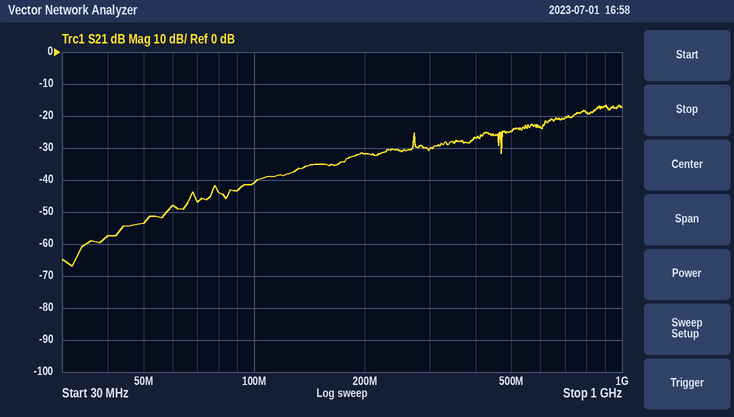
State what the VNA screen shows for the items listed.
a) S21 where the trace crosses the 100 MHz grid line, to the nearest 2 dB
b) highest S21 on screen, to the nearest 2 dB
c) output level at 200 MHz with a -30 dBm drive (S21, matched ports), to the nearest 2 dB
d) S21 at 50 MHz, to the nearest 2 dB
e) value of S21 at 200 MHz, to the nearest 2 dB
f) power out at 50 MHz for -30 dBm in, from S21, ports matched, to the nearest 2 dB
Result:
-40 dB
-16 dB
-62 dBm
-54 dB
-32 dB
-84 dBm
